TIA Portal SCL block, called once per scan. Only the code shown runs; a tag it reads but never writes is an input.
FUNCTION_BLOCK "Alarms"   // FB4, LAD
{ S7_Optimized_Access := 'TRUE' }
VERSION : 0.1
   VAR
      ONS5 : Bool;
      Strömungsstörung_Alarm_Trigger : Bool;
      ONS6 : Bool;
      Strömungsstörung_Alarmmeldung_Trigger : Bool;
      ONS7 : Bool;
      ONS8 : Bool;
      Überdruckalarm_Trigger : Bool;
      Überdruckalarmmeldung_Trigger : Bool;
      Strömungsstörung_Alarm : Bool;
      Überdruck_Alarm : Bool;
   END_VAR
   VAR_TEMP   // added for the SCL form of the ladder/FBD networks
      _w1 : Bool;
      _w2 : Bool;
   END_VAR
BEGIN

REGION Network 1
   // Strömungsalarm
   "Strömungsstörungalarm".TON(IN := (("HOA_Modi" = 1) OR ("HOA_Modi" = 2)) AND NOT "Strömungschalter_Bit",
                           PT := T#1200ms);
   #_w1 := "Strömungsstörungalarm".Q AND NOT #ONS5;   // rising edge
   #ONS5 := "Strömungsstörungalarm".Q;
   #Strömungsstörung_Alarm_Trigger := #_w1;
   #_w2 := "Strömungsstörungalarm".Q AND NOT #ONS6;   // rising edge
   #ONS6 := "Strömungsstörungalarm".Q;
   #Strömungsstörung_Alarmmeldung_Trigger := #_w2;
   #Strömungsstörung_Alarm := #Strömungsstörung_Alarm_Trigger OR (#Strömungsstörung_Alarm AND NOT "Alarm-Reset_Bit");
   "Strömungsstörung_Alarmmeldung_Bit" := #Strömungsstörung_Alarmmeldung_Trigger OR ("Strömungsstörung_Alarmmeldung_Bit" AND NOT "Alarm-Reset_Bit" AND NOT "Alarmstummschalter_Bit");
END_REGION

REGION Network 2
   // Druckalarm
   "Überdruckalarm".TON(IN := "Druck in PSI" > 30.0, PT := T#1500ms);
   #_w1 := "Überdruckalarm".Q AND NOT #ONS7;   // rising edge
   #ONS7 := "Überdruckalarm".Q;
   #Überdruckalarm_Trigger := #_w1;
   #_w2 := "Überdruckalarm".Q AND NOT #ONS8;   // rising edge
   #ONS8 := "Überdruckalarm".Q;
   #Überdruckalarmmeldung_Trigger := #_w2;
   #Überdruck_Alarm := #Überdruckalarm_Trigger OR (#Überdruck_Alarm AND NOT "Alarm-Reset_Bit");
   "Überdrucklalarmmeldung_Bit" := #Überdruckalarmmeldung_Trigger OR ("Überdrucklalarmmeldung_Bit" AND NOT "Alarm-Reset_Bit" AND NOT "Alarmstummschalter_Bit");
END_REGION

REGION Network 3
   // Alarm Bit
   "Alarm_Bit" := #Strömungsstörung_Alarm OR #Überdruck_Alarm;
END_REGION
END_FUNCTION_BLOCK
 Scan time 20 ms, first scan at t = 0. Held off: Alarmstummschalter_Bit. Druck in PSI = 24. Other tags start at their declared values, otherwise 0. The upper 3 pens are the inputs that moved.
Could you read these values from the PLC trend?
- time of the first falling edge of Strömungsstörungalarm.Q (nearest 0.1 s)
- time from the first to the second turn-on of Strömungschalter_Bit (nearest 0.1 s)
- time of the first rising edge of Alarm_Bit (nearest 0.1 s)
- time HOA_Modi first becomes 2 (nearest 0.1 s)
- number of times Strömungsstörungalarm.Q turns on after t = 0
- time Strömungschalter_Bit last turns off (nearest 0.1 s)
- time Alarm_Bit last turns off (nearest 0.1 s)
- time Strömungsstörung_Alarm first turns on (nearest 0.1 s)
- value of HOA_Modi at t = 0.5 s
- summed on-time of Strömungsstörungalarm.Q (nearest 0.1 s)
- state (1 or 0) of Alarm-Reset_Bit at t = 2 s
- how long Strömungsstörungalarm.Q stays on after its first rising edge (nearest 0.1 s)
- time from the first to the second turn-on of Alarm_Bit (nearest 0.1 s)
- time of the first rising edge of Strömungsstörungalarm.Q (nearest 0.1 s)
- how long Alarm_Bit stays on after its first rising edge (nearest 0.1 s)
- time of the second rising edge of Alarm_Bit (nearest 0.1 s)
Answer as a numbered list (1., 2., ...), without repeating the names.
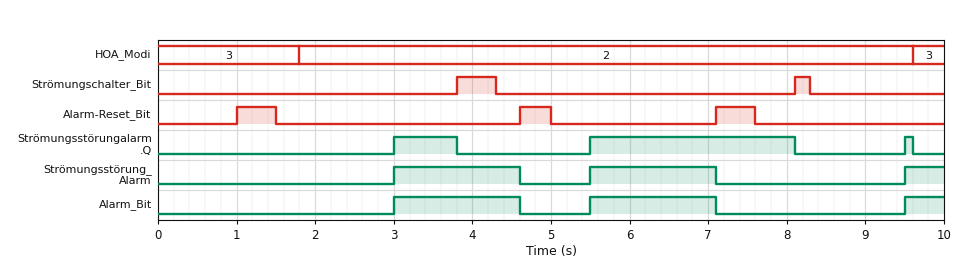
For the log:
1. 3.8 s
2. 4.3 s
3. 3.0 s
4. 1.8 s
5. 3
6. 8.3 s
7. 7.1 s
8. 3.0 s
9. 3
10. 3.5 s
11. 0
12. 0.8 s
13. 2.5 s
14. 3.0 s
15. 1.6 s
16. 5.5 s
